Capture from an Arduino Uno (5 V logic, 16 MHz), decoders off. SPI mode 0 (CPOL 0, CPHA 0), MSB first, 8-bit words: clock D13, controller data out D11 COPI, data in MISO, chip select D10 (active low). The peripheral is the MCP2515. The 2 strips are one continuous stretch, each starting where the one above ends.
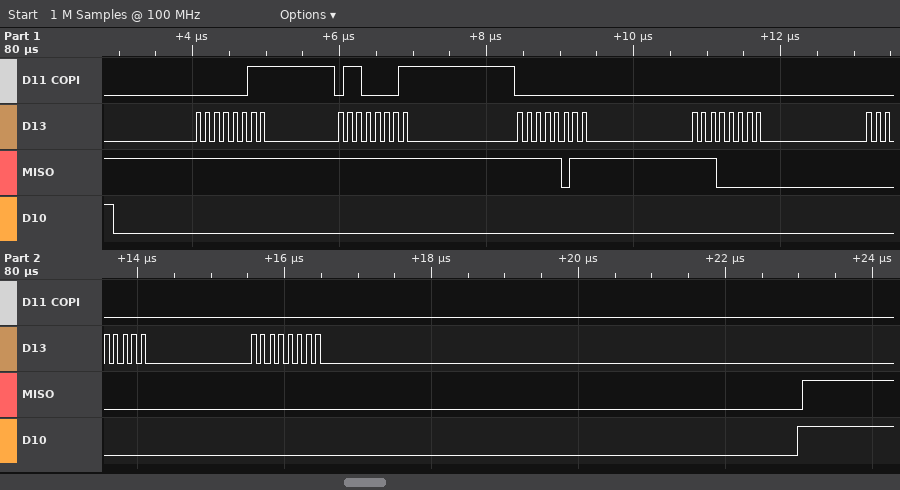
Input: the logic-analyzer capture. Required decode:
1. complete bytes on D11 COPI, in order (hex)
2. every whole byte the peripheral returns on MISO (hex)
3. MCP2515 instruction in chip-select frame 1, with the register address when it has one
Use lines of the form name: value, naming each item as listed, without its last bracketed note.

complete bytes on D11 COPI, in order: 03 61 00 00 00 00
every whole byte the peripheral returns on MISO: FF FF FB E0 00 00
MCP2515 instruction in chip-select frame 1, with the register address when it has one: READ 0x61
